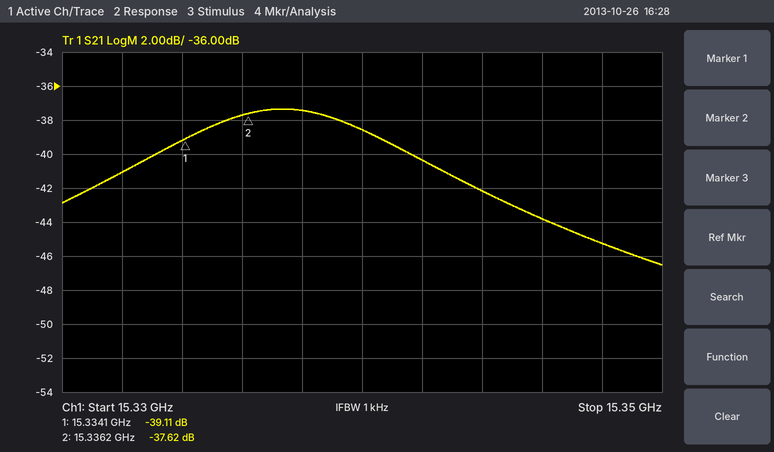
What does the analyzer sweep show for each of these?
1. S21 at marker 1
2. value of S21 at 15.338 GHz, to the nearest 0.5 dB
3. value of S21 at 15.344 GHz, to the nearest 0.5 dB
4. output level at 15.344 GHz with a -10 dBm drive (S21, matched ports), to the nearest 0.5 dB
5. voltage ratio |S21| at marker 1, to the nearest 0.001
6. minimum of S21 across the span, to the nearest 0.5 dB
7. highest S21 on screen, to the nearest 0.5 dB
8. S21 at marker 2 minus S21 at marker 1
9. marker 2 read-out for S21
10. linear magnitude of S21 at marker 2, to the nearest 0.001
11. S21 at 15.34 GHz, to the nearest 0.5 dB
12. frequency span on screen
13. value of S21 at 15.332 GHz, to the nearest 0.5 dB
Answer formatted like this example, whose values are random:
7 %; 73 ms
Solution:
-39.11 dB; -37.5 dB; -42.0 dB; -52.0 dBm; 0.011; -46.5 dB; -37.5 dB; 1.49 dB; -37.62 dB; 0.013; -38.5 dB; 20 MHz; -41.0 dB
